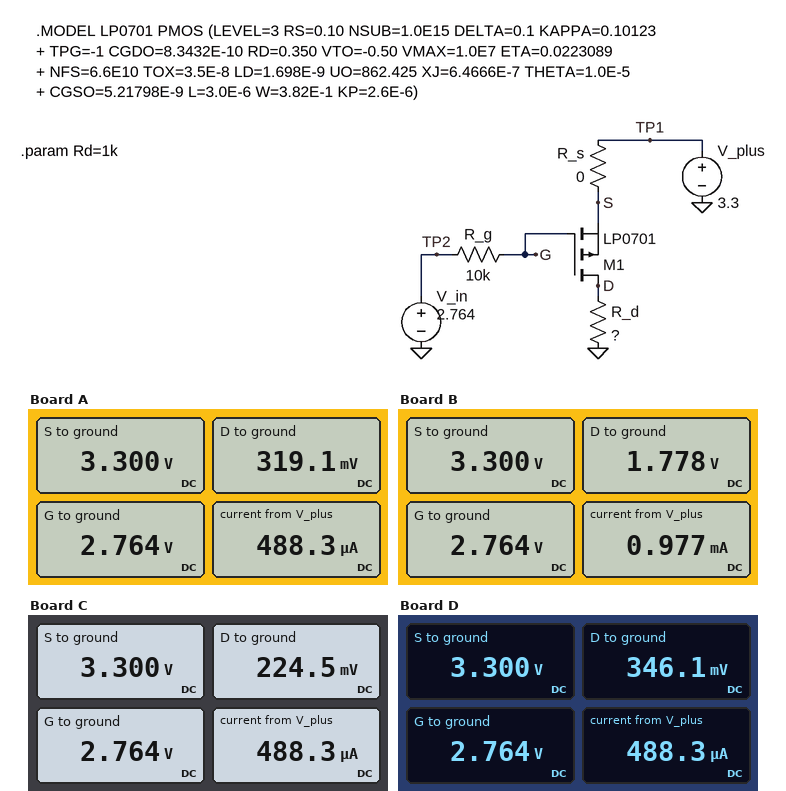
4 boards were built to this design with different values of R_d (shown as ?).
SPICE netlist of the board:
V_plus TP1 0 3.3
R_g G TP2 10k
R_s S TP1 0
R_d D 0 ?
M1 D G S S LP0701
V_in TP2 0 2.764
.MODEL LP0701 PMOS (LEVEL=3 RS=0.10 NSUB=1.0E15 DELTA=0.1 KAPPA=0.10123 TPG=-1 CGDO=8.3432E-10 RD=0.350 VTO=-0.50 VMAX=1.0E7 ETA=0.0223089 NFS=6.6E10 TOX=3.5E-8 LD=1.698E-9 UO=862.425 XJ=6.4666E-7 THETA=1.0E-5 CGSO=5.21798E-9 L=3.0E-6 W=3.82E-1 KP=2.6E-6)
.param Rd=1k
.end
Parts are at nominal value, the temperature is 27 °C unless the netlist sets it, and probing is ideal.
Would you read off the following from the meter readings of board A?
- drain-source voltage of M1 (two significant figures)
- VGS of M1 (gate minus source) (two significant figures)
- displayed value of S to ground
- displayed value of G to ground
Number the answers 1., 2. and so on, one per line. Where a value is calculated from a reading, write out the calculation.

1. 319.1 mV - 3.3 V = -3.0 V
2. 2.764 V - 3.3 V = -540 mV
3. 3.300 V
4. 2.764 V
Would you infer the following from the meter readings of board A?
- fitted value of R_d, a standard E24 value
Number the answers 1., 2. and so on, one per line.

1. 470 Ω
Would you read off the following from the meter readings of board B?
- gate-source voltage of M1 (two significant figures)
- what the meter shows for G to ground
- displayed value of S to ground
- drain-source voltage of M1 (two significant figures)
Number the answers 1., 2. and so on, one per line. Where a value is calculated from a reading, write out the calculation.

1. 2.764 V - 3.3 V = -540 mV
2. 2.764 V
3. 3.300 V
4. 1.778 V - 3.3 V = -1.5 V
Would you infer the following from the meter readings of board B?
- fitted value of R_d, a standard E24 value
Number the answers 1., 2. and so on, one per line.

1. 2.7 kΩ
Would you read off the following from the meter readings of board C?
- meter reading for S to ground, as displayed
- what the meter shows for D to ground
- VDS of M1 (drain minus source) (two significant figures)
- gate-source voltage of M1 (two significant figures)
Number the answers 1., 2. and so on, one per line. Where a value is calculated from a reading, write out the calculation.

1. 3.300 V
2. 224.5 mV
3. 224.5 mV - 3.3 V = -3.1 V
4. 2.764 V - 3.3 V = -540 mV
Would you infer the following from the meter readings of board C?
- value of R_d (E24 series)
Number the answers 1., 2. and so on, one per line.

1. 330 Ω
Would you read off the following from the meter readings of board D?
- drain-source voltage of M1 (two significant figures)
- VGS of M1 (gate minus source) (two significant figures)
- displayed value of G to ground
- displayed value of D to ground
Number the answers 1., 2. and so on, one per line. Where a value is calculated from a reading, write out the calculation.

1. 346.1 mV - 3.3 V = -3.0 V
2. 2.764 V - 3.3 V = -540 mV
3. 2.764 V
4. 346.1 mV
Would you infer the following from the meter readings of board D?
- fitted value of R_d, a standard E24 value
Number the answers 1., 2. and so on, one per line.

1. 510 Ω
